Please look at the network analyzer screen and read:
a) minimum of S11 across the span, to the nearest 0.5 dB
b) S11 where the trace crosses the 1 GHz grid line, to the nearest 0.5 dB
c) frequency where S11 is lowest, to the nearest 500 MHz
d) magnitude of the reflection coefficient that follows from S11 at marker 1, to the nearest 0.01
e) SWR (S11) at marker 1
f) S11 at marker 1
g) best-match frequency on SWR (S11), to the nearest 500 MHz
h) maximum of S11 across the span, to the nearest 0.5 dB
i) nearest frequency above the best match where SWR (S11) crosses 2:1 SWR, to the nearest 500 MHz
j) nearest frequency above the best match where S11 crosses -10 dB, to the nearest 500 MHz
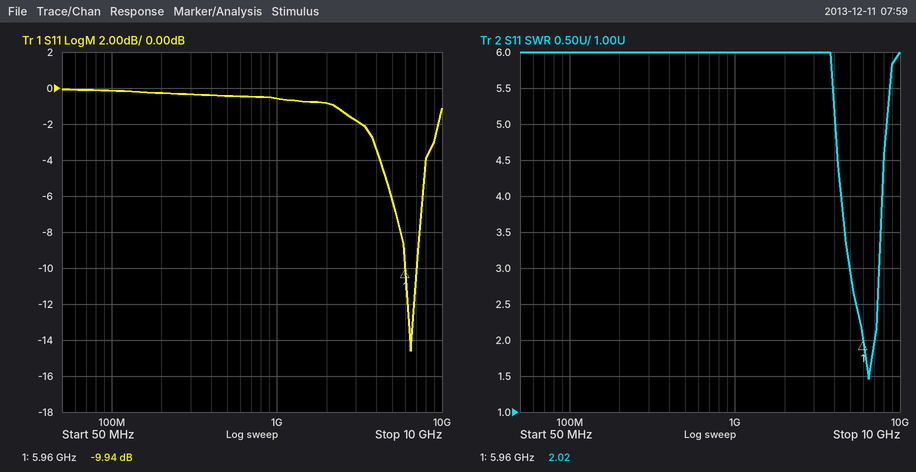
-14.5 dB
-0.5 dB
6.5 GHz
0.32
2.02
-9.94 dB
6.5 GHz
0.0 dB
7.0 GHz
7.0 GHz
